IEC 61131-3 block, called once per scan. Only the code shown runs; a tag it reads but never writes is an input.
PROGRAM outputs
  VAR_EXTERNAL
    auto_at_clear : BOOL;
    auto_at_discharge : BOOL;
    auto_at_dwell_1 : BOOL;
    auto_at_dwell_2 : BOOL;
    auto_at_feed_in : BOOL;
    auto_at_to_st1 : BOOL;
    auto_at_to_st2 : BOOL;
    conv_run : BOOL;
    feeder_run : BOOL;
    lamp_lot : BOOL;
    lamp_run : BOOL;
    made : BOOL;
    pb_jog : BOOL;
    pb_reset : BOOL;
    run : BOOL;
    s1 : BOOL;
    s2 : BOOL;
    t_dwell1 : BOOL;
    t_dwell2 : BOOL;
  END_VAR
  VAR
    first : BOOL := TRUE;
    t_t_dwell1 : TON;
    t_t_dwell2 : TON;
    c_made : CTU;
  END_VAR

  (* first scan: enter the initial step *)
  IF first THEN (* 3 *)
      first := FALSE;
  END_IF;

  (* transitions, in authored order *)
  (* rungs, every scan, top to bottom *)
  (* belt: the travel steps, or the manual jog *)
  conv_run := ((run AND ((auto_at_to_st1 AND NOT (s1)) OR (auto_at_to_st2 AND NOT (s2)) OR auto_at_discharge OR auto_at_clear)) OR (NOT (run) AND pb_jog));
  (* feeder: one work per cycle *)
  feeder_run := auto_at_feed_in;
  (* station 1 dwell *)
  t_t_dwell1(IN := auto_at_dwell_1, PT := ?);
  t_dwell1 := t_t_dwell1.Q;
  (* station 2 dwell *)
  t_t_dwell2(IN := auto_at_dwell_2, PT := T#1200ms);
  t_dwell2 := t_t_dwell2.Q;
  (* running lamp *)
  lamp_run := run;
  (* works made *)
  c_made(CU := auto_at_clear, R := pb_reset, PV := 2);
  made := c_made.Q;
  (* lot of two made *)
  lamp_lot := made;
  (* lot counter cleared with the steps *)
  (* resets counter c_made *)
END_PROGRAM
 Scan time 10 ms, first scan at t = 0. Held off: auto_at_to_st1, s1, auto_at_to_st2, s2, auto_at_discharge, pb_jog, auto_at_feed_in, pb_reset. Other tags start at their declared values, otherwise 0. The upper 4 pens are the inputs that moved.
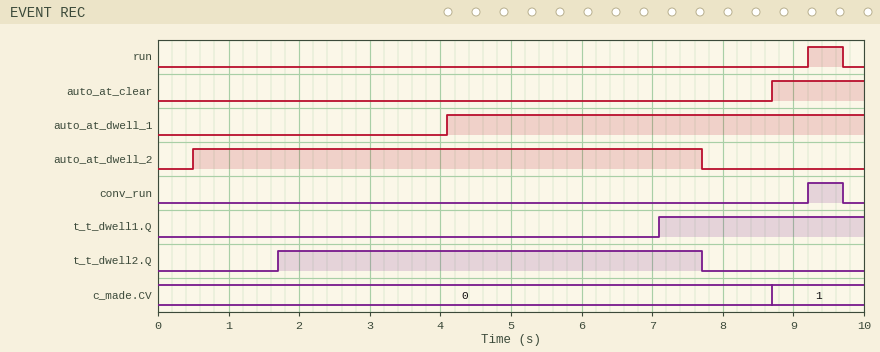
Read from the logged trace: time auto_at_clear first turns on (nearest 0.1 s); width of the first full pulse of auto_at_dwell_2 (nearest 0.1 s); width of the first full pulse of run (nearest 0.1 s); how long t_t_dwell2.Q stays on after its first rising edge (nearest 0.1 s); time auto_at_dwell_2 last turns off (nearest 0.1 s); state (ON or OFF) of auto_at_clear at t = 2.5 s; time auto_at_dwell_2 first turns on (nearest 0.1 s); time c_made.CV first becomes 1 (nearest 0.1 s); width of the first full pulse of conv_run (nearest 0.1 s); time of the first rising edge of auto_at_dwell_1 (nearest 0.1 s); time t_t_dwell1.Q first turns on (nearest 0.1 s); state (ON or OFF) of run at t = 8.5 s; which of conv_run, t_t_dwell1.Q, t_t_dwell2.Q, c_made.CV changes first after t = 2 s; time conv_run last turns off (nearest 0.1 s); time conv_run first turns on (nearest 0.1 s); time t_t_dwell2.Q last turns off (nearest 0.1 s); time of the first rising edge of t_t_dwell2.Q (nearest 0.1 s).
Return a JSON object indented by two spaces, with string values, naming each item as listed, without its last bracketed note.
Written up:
{
  "time auto_at_clear first turns on": "8.7 s",
  "width of the first full pulse of auto_at_dwell_2": "7.2 s",
  "width of the first full pulse of run": "0.5 s",
  "how long t_t_dwell2.Q stays on after its first rising edge": "6.0 s",
  "time auto_at_dwell_2 last turns off": "7.7 s",
  "state (ON or OFF) of auto_at_clear at t = 2.5 s": "OFF",
  "time auto_at_dwell_2 first turns on": "0.5 s",
  "time c_made.CV first becomes 1": "8.7 s",
  "width of the first full pulse of conv_run": "0.5 s",
  "time of the first rising edge of auto_at_dwell_1": "4.1 s",
  "time t_t_dwell1.Q first turns on": "7.1 s",
  "state (ON or OFF) of run at t = 8.5 s": "OFF",
  "which of conv_run, t_t_dwell1.Q, t_t_dwell2.Q, c_made.CV changes first after t = 2 s": "t_t_dwell1.Q",
  "time conv_run last turns off": "9.7 s",
  "time conv_run first turns on": "9.2 s",
  "time t_t_dwell2.Q last turns off": "7.7 s",
  "time of the first rising edge of t_t_dwell2.Q": "1.7 s"
}
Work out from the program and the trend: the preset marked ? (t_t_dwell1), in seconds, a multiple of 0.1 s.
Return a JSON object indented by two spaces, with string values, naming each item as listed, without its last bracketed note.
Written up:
{
  "the preset marked ? (t_t_dwell1), in seconds, a multiple of 0.1 s": "3.0 s"
}
